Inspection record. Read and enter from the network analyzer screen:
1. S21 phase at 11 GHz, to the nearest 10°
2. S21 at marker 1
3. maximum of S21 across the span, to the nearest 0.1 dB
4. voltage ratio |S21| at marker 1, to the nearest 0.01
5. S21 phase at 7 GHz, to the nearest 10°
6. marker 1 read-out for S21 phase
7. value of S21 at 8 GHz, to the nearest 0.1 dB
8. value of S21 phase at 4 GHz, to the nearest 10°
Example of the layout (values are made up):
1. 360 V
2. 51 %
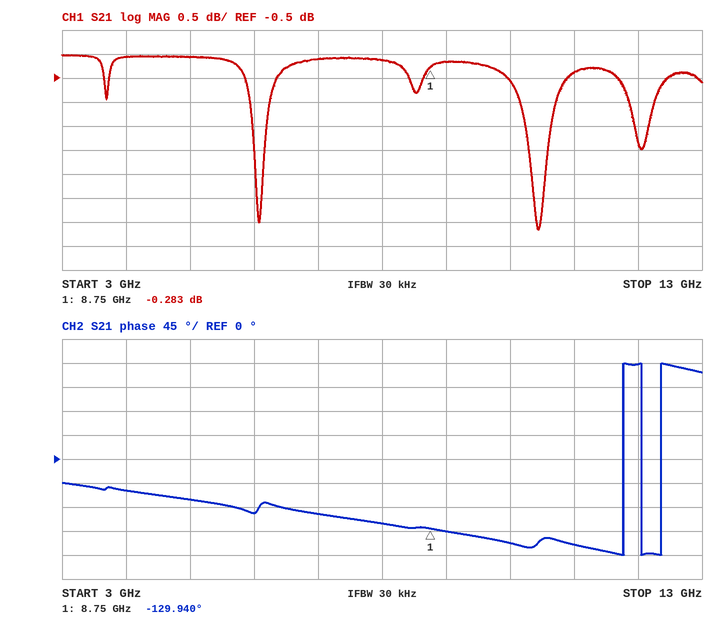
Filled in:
1. -160°
2. -0.283 dB
3. 0.0 dB
4. 0.97
5. -100°
6. -129.940°
7. -0.1 dB
8. -60°
